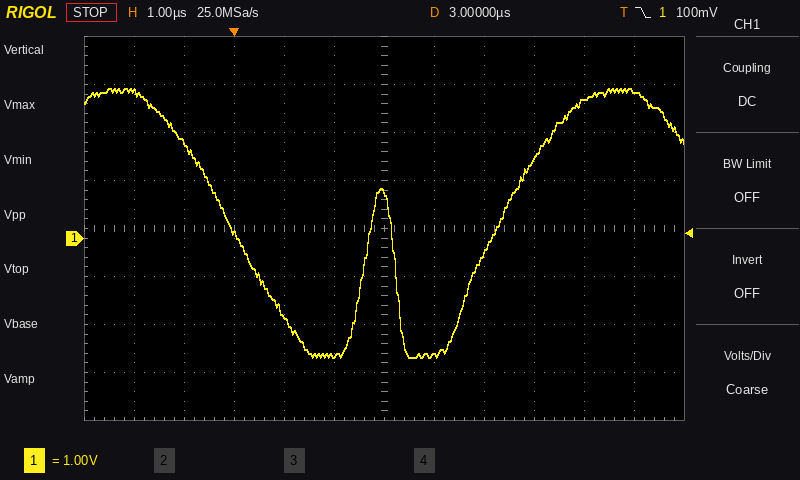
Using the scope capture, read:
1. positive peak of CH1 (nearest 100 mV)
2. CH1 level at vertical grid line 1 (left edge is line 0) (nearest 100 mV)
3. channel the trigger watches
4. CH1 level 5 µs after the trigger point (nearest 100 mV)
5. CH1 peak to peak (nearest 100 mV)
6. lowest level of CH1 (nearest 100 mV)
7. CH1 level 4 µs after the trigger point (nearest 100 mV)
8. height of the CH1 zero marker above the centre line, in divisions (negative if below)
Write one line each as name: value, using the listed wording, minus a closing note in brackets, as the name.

positive peak of CH1: 3.1 V
CH1 level at vertical grid line 1 (left edge is line 0): 3.0 V
channel the trigger watches: CH1
CH1 level 5 µs after the trigger point: -300 mV
CH1 peak to peak: 5.6 V
lowest level of CH1: -2.5 V
CH1 level 4 µs after the trigger point: -2.4 V
height of the CH1 zero marker above the centre line, in divisions: -0.2 div
